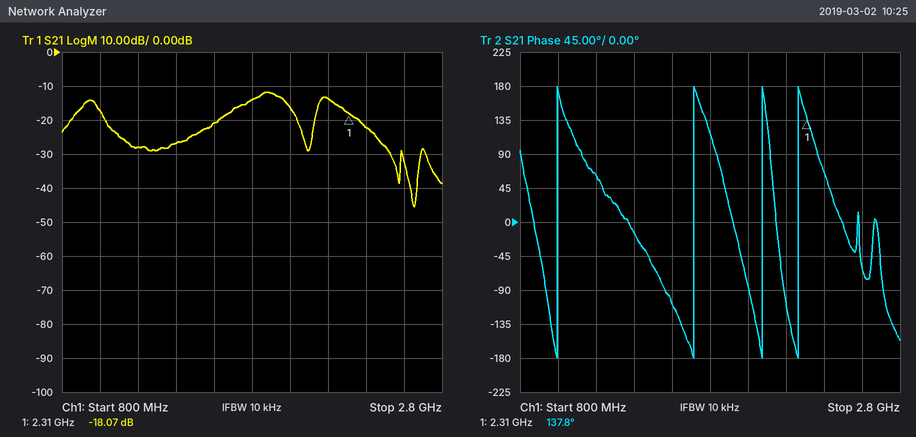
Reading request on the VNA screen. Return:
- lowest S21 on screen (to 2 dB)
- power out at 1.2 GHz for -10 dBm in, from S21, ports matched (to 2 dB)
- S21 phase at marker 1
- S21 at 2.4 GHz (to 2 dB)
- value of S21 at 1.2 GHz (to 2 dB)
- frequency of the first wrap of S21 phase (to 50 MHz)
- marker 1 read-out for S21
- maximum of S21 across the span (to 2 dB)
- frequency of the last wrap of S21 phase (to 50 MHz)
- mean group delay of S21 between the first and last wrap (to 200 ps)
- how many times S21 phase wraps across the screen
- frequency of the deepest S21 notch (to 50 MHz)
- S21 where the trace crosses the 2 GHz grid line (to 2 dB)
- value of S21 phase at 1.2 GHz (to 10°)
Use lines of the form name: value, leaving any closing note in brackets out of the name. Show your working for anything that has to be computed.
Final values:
lowest S21 on screen: -46 dB
power out at 1.2 GHz for -10 dBm in, from S21, ports matched: -10 dBm + (-28 dB) = -38 dBm
S21 phase at marker 1: 137.8°
S21 at 2.4 GHz: -22 dB
value of S21 at 1.2 GHz: -28 dB
frequency of the first wrap of S21 phase: 1.00 GHz
marker 1 read-out for S21: -18.07 dB
maximum of S21 across the span: -12 dB
frequency of the last wrap of S21 phase: 2.25 GHz
mean group delay of S21 between the first and last wrap: 3 cycles / (2.25 GHz − 1.00 GHz) ≈ 2.4 ns
how many times S21 phase wraps across the screen: 4
frequency of the deepest S21 notch: 2.65 GHz
S21 where the trace crosses the 2 GHz grid line: -16 dB
value of S21 phase at 1.2 GHz: 60°
